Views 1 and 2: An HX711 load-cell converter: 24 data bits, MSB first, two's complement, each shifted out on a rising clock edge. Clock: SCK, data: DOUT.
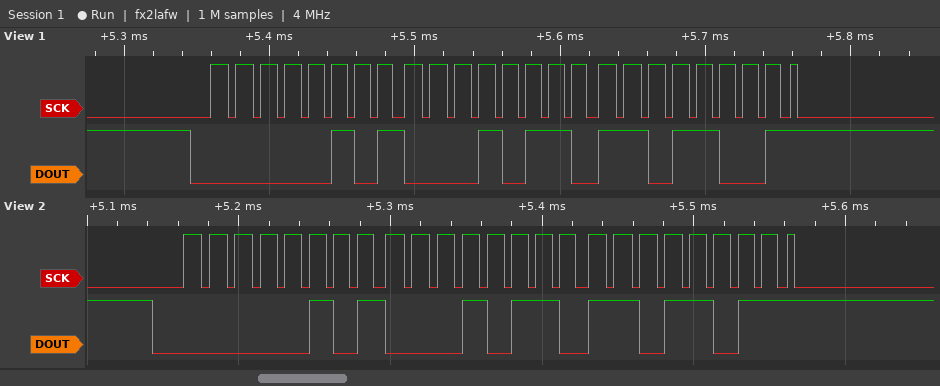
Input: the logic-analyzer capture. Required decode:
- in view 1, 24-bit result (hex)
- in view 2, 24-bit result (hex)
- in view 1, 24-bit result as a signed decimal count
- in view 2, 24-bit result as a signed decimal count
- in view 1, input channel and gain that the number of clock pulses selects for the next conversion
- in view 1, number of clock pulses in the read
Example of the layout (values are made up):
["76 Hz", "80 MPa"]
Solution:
["0x0516D9", "0x0516DB", "333529", "333531", "channel A, gain 128", "25"]
